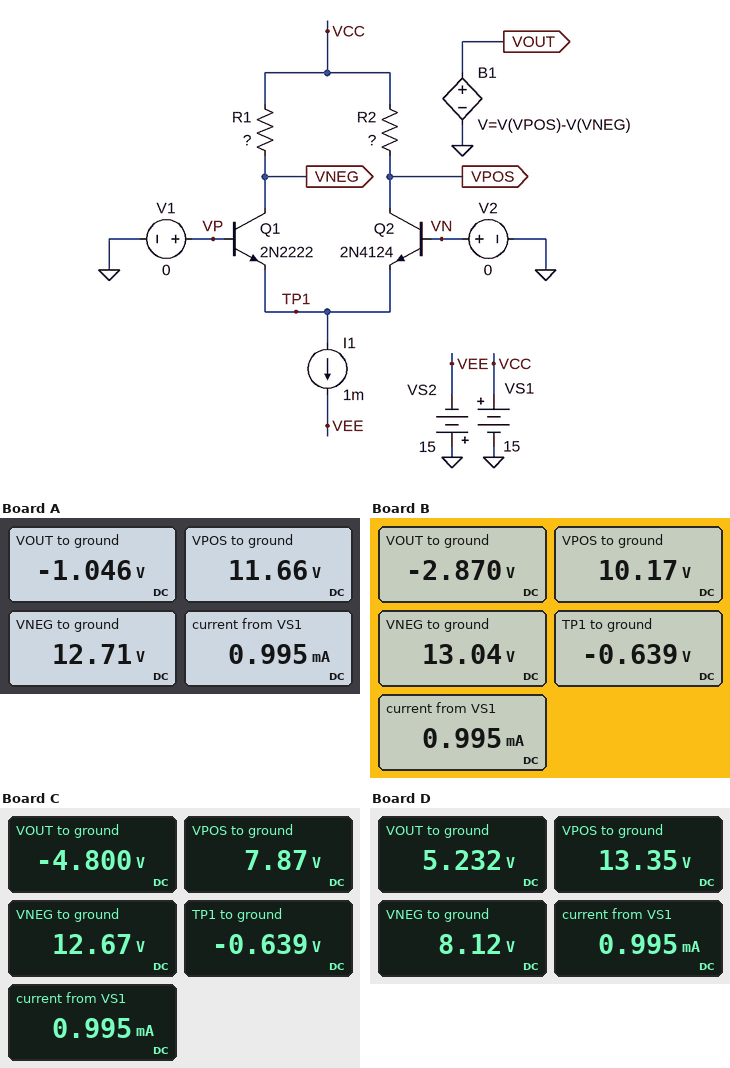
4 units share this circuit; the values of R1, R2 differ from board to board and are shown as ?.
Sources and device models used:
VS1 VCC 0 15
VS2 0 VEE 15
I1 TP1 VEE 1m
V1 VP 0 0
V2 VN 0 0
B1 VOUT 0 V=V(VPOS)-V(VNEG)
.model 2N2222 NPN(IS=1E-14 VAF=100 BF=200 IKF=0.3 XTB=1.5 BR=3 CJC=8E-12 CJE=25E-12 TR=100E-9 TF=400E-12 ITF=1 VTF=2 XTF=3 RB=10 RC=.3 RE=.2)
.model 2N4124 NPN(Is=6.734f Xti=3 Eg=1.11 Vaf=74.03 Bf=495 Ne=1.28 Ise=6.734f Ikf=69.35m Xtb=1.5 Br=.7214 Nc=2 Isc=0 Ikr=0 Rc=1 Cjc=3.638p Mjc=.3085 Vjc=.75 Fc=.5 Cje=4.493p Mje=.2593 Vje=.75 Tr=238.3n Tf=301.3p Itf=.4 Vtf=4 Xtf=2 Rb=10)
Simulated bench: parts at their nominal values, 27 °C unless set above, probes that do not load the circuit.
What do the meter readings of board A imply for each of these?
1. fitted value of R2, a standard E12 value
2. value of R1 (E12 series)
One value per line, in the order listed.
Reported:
8.2 kΩ
3.9 kΩ
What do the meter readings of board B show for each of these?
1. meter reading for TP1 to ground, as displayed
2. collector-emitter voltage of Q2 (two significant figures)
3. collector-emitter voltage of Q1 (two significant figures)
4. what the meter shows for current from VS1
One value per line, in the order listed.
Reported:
-0.639 V
11 V
14 V
0.995 mA
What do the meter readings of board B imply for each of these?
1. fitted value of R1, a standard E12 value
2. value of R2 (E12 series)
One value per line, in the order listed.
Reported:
3.3 kΩ
12 kΩ
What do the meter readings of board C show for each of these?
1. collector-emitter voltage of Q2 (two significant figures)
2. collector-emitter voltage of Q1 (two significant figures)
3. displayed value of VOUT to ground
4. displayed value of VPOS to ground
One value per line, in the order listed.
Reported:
8.5 V
13 V
-4.800 V
7.87 V
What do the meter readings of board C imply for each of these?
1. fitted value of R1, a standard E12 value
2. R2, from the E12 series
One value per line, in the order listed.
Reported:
3.9 kΩ
18 kΩ
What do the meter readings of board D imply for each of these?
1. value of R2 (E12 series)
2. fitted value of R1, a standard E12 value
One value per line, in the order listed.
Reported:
3.9 kΩ
12 kΩ
